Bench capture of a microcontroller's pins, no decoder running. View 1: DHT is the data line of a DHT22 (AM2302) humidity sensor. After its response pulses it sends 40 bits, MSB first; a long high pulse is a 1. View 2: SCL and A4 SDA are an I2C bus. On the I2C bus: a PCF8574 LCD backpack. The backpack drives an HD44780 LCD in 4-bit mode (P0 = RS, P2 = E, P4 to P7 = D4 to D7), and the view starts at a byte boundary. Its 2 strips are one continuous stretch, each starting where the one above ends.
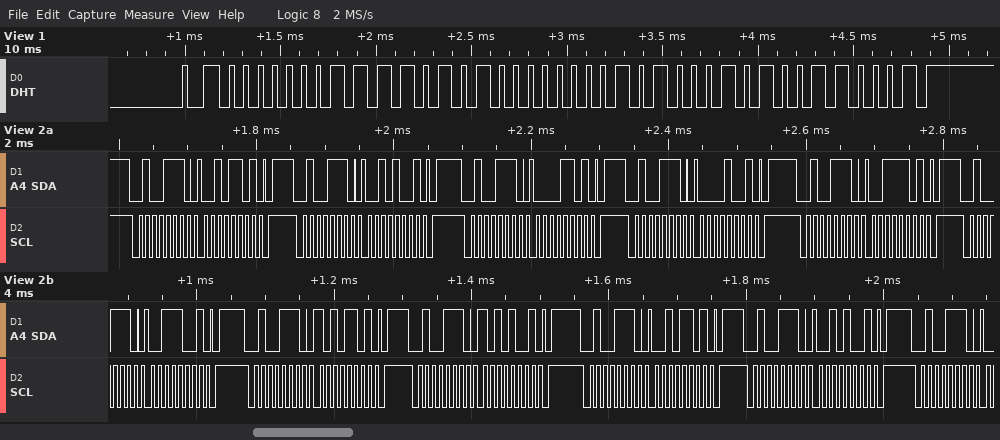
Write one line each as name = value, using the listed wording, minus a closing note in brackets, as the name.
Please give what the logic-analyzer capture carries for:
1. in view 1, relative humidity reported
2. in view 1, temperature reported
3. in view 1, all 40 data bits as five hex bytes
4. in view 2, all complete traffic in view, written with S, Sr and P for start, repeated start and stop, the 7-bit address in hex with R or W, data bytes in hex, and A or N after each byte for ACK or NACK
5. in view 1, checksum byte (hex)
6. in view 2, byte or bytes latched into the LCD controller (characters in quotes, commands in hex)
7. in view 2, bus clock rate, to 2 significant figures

in view 1, relative humidity reported = 49.0 %
in view 1, temperature reported = 32.5 °C
in view 1, all 40 data bits as five hex bytes = 01 EA 01 45 31
in view 2, all complete traffic in view, written with S, Sr and P for start, repeated start and stop, the 7-bit address in hex with R or W, data bytes in hex, and A or N after each byte for ACK or NACK = S 27W A 2D A P S 27W A 29 A P S 27W A 0D A P S 27W A 09 A P S 27W A 3D A P S 27W A 39 A P S 27W A AD A P S 27W A A9 A P S 27W A 2D A P S 27W A 29 A P S 27W A
in view 1, checksum byte = 0x31
in view 2, byte or bytes latched into the LCD controller = ' ' ':'
in view 2, bus clock rate, to 2 significant figures = 100 kHz
